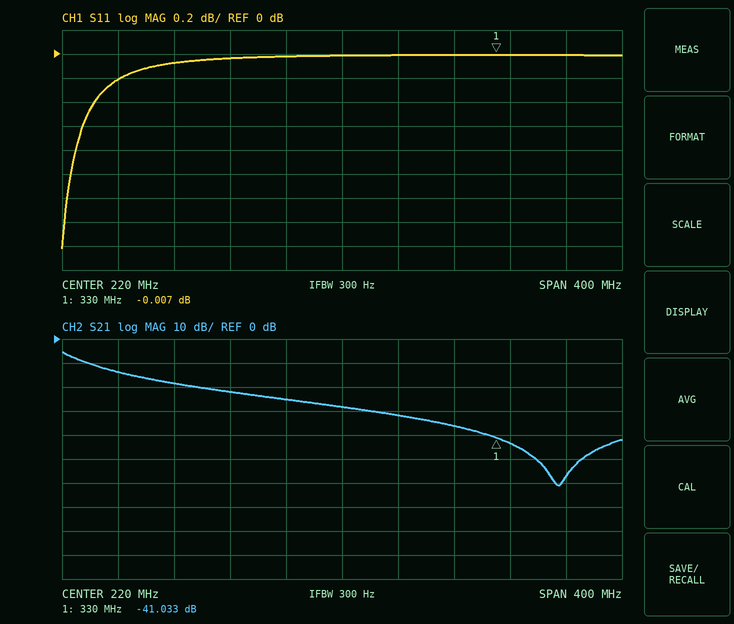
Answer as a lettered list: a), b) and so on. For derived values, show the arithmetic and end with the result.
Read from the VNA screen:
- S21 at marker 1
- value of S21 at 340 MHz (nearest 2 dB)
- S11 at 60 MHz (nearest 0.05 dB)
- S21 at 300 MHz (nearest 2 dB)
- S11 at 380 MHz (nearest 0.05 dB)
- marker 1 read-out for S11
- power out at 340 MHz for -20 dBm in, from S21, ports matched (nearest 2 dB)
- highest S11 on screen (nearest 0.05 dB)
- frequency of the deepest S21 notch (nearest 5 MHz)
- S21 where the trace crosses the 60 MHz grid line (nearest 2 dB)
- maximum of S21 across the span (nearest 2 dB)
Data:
a) -41.033 dB
b) -44 dB
c) -0.20 dB
d) -36 dB
e) 0.00 dB
f) -0.007 dB
g) -20 dBm + (-44 dB) = -64 dBm
h) 0.00 dB
i) 375 MHz
j) -14 dB
k) -6 dB
